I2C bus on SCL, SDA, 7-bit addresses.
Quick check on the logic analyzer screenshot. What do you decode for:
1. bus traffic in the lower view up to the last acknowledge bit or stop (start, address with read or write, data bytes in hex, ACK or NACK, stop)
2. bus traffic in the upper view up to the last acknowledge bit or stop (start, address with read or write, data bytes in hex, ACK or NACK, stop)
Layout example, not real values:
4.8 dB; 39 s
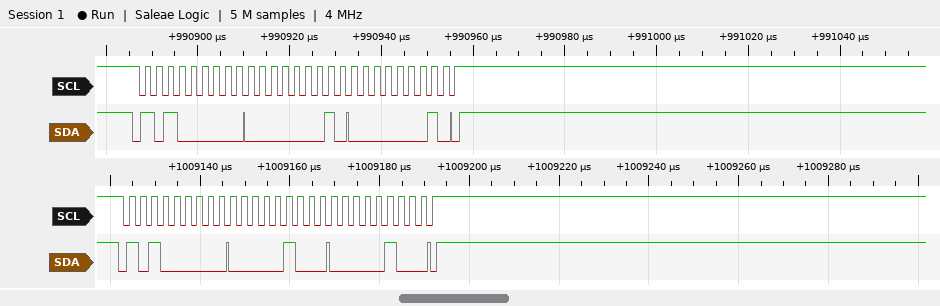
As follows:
start, address 50 write ACK, 04 ACK, 04 ACK, stop; start, address 50 write ACK, 01 ACK, 01 ACK, stop
